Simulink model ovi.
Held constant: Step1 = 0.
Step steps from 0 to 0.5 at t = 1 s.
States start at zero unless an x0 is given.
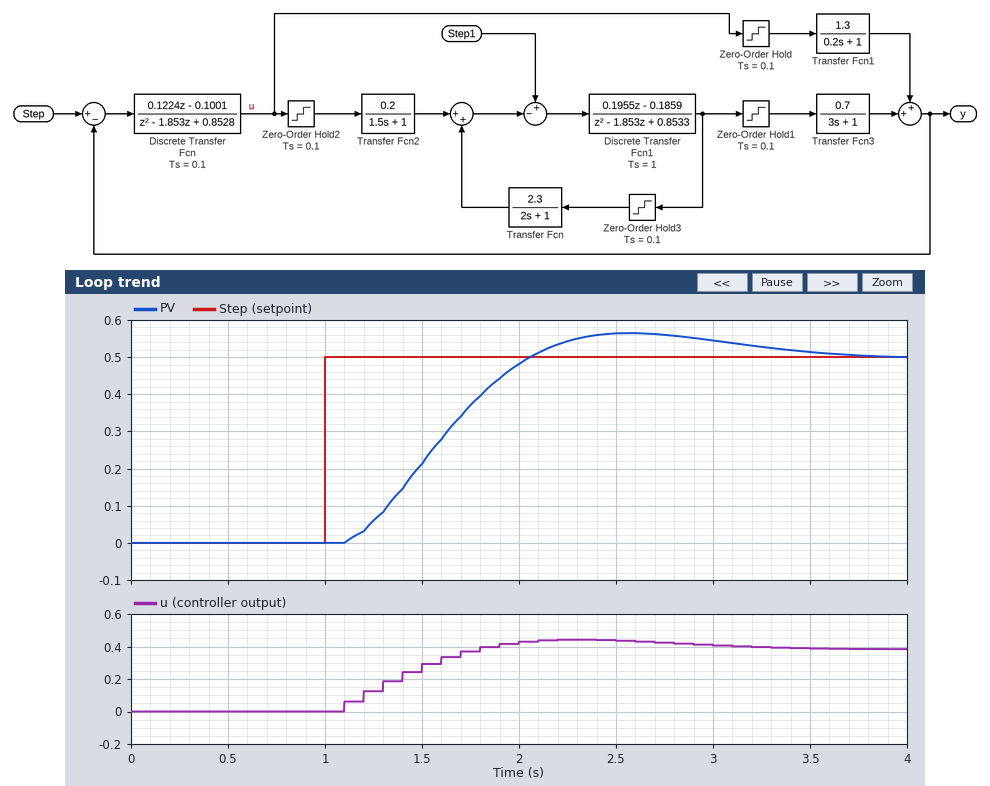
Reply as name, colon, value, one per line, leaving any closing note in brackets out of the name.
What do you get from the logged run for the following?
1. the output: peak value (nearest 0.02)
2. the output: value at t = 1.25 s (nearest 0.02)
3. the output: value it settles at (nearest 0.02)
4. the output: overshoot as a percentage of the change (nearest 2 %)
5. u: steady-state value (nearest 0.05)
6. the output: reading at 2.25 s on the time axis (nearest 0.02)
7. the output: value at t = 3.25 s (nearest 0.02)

the output: peak value: 0.56
the output: value at t = 1.25 s: 0.06
the output: value it settles at: 0.50
the output: overshoot as a percentage of the change: 12 %
u: steady-state value: 0.40
the output: reading at 2.25 s on the time axis: 0.54
the output: value at t = 3.25 s: 0.52
